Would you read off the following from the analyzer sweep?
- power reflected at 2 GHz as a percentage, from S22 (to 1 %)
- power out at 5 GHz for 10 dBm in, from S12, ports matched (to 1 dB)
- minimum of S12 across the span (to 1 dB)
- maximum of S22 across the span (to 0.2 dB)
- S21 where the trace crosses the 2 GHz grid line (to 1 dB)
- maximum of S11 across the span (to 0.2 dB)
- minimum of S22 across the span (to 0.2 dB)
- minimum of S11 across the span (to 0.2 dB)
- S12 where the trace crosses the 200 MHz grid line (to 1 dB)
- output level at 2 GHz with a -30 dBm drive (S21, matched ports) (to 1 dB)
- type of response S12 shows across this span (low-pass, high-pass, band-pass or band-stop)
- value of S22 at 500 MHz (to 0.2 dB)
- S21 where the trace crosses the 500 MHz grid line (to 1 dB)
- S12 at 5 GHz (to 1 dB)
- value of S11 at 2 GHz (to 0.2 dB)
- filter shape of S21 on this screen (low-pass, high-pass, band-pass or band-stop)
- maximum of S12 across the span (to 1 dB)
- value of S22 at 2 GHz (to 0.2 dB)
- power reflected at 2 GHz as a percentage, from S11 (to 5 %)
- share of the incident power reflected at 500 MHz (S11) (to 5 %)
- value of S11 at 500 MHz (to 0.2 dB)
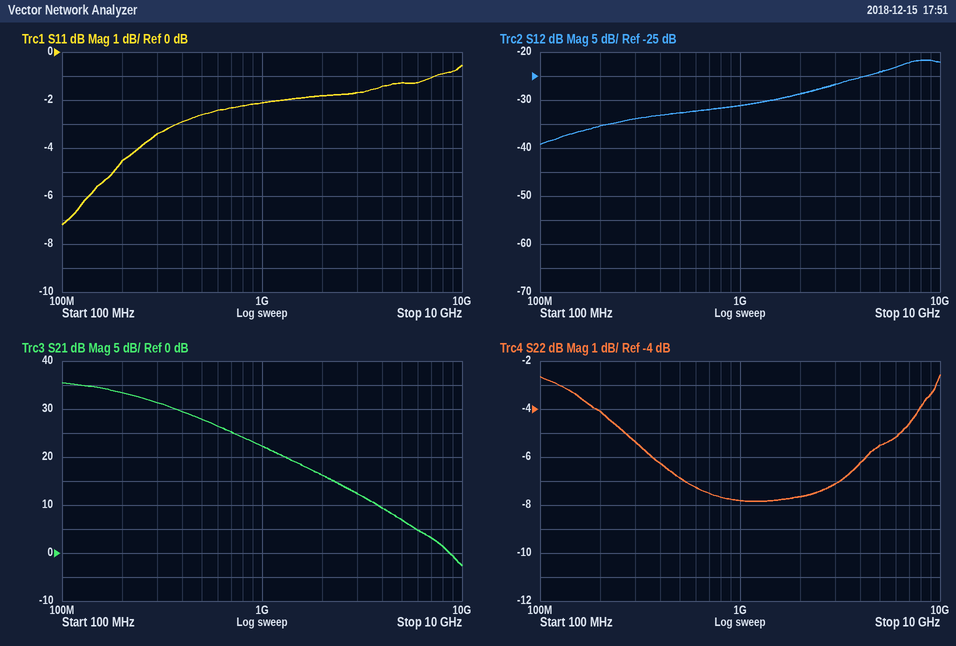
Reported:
17 %
-14 dBm
-39 dB
-2.6 dB
16 dB
-0.6 dB
-7.8 dB
-7.2 dB
-35 dB
-14 dBm
high-pass
-6.8 dB
28 dB
-24 dB
-1.8 dB
low-pass
-22 dB
-7.6 dB
65 %
55 %
-2.6 dB
